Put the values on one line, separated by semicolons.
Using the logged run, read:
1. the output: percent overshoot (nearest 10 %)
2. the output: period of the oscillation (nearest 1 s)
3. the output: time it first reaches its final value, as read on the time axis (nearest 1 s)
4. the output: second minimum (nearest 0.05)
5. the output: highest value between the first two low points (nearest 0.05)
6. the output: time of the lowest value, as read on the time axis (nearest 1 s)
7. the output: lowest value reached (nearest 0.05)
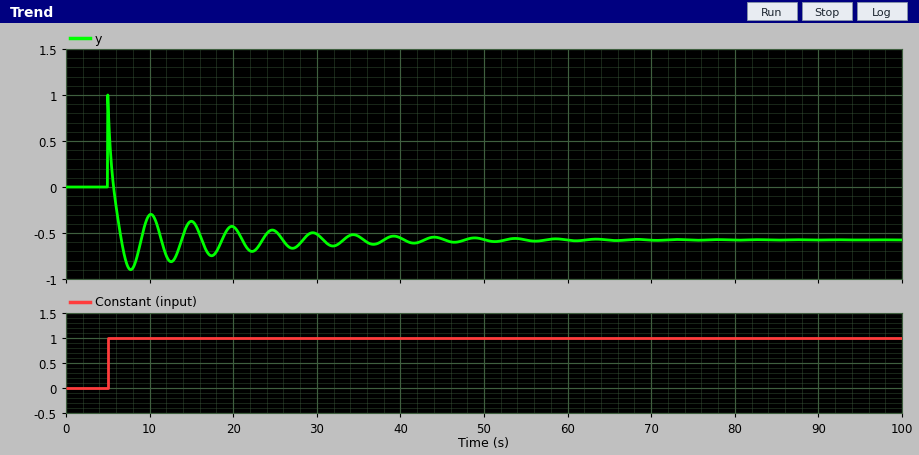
60 %; 5 s; 7 s; -0.80; -0.30; 8 s; -0.90
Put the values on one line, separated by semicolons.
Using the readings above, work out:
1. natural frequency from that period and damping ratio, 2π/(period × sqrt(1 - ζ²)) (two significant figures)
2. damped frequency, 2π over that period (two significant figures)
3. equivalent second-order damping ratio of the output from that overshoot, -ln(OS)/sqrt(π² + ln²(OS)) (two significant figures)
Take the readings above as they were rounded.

1.3 rad/s; 1.3 rad/s; 0.16
